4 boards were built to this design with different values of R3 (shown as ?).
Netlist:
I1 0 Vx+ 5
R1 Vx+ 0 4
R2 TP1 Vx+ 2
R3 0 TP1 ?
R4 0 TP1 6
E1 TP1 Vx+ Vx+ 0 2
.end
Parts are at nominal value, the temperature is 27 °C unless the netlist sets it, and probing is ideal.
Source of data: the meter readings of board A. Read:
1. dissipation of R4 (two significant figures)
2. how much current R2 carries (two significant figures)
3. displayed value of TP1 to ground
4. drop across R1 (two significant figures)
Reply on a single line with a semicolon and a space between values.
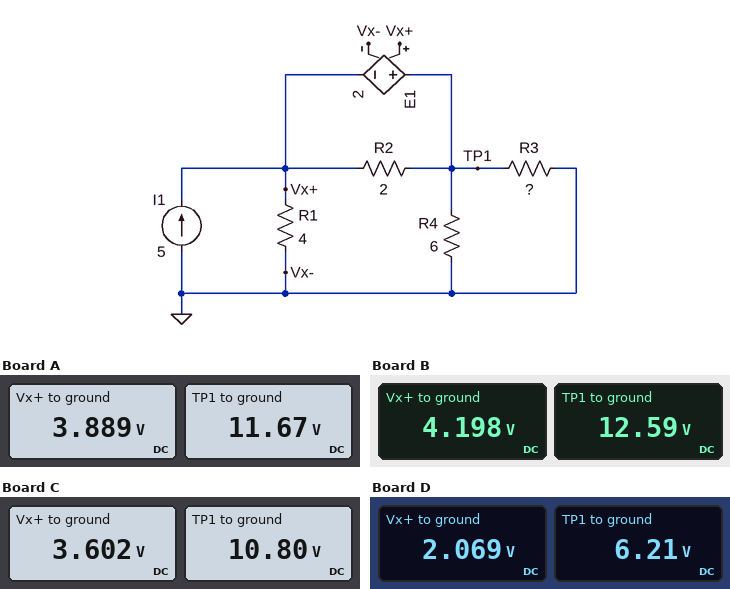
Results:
23 W; 3.9 A; 11.67 V; 3.9 V
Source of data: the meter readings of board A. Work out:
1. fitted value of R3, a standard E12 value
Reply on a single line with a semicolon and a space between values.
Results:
5.6 Ω
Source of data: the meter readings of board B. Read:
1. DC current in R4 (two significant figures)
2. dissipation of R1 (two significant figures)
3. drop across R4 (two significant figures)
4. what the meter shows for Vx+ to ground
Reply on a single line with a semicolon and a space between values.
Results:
2.1 A; 4.4 W; 13 V; 4.198 V
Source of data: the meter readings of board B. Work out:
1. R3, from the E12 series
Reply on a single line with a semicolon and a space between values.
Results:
6.8 Ω
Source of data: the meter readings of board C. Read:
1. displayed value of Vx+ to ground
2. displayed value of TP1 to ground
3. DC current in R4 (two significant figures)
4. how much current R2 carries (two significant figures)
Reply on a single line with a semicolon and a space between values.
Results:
3.602 V; 10.80 V; 1.8 A; 3.6 A
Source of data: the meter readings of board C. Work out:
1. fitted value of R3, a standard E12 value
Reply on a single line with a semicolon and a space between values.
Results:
4.7 Ω
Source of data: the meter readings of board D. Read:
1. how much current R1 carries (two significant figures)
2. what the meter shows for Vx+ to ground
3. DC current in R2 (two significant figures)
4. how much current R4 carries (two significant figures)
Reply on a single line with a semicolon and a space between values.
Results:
520 mA; 2.069 V; 2.1 A; 1.0 A
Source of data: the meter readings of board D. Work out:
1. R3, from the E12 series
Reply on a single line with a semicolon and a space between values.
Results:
1.8 Ω
